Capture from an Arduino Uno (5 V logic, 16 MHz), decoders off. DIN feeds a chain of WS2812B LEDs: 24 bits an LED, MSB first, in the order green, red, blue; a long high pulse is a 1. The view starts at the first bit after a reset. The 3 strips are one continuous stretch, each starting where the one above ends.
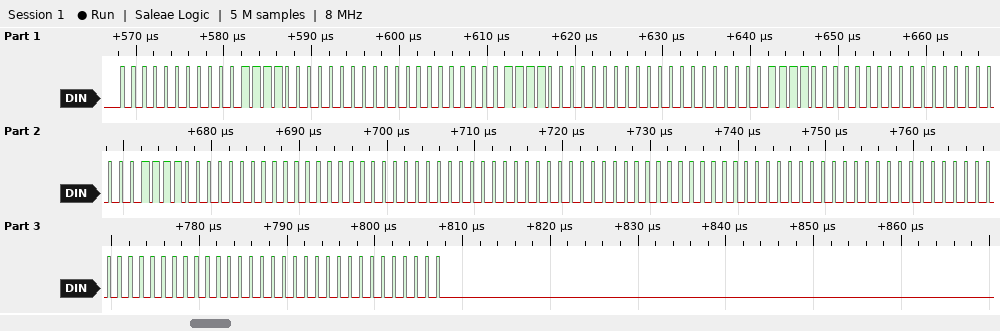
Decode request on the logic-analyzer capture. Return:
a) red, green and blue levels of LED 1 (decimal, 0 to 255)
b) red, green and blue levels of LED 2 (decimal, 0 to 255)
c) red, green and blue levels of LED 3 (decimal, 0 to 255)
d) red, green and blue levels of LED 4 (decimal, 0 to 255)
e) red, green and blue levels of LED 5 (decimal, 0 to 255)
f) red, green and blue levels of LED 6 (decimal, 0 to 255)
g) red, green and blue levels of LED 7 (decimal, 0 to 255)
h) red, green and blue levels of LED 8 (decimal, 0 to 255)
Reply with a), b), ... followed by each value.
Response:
a) 30, 0, 0
b) 30, 0, 0
c) 30, 0, 0
d) 30, 0, 0
e) 0, 0, 0
f) 0, 0, 0
g) 0, 0, 0
h) 0, 0, 0
